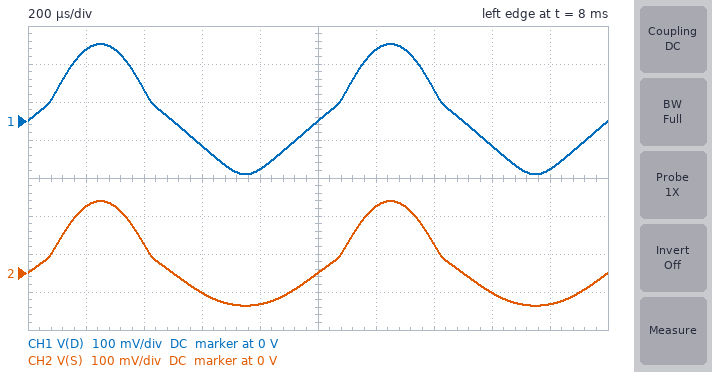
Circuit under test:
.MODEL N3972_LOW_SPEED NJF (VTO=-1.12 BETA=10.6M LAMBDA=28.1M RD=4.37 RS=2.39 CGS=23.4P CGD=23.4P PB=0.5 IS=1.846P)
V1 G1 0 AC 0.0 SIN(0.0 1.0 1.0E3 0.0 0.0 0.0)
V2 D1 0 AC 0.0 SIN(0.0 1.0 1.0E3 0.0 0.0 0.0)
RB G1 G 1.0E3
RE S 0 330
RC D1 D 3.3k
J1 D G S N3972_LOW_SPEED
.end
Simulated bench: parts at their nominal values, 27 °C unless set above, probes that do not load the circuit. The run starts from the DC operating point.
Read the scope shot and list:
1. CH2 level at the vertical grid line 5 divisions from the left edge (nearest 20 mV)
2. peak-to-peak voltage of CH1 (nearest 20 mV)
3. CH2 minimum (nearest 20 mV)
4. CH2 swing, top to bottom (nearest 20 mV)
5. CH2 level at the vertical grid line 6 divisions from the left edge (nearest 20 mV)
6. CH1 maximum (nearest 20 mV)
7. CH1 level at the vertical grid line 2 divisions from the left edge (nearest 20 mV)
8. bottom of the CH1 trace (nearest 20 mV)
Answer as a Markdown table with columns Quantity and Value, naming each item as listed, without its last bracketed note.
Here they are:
| Quantity | Value |
|---|---|
| CH2 level at the vertical grid line 5 divisions from the left edge | 0 V |
| peak-to-peak voltage of CH1 | 340 mV |
| CH2 minimum | -80 mV |
| CH2 swing, top to bottom | 280 mV |
| CH2 level at the vertical grid line 6 divisions from the left edge | 180 mV |
| CH1 maximum | 200 mV |
| CH1 level at the vertical grid line 2 divisions from the left edge | 80 mV |
| bottom of the CH1 trace | -140 mV |
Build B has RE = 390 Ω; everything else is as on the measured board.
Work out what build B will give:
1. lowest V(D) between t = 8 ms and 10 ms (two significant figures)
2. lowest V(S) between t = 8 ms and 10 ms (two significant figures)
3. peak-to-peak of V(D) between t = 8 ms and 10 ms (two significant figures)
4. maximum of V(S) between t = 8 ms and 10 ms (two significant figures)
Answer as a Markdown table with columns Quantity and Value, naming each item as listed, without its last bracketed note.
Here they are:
| Quantity | Value |
|---|---|
| lowest V(D) between t = 8 ms and 10 ms | -150 mV |
| lowest V(S) between t = 8 ms and 10 ms | -100 mV |
| peak-to-peak of V(D) between t = 8 ms and 10 ms | 380 mV |
| maximum of V(S) between t = 8 ms and 10 ms | 210 mV |
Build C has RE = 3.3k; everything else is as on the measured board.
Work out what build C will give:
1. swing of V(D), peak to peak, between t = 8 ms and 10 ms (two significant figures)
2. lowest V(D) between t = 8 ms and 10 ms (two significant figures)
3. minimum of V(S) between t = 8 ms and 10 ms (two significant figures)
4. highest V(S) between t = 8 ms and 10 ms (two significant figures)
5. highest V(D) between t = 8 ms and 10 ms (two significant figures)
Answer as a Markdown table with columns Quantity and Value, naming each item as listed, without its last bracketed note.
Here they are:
| Quantity | Value |
|---|---|
| swing of V(D), peak to peak, between t = 8 ms and 10 ms | 1.1 V |
| lowest V(D) between t = 8 ms and 10 ms | -510 mV |
| minimum of V(S) between t = 8 ms and 10 ms | -490 mV |
| highest V(S) between t = 8 ms and 10 ms | 550 mV |
| highest V(D) between t = 8 ms and 10 ms | 560 mV |
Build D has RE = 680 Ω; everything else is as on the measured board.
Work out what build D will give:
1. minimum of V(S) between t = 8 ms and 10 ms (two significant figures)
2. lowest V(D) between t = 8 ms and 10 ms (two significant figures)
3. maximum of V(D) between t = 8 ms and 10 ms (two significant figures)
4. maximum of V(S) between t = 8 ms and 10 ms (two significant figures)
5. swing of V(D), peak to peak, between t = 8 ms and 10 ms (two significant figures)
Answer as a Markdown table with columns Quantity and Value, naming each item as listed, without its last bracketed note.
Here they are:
| Quantity | Value |
|---|---|
| minimum of V(S) between t = 8 ms and 10 ms | -160 mV |
| lowest V(D) between t = 8 ms and 10 ms | -200 mV |
| maximum of V(D) between t = 8 ms and 10 ms | 310 mV |
| maximum of V(S) between t = 8 ms and 10 ms | 300 mV |
| swing of V(D), peak to peak, between t = 8 ms and 10 ms | 510 mV |
